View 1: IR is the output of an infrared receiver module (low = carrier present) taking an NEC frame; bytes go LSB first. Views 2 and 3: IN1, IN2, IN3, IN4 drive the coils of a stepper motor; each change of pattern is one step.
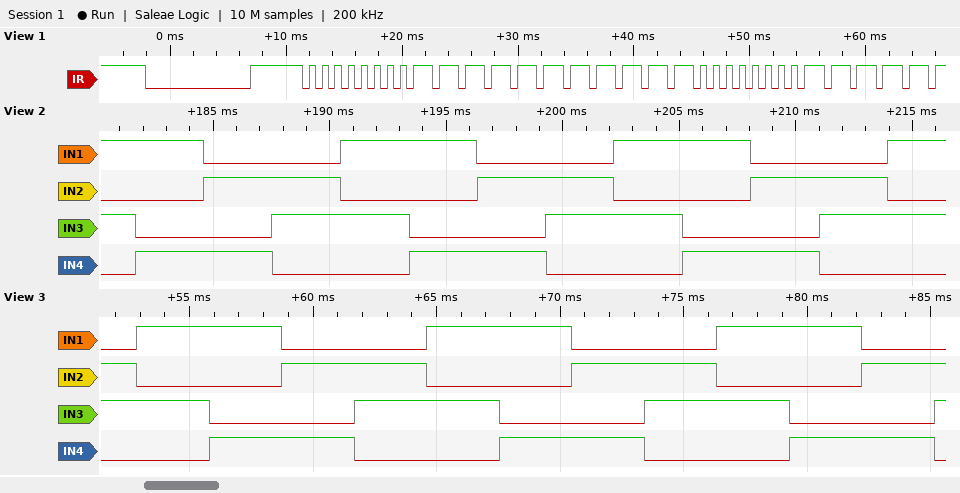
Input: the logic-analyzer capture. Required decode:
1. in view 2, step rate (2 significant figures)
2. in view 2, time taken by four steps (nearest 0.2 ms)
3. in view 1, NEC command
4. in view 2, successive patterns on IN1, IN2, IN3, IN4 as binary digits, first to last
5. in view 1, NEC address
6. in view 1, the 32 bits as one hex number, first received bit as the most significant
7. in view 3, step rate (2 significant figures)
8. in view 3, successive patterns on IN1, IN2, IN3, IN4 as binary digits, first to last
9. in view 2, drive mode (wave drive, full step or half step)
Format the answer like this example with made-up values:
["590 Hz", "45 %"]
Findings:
["340 steps/s", "11.8 ms", "0x07", "1010 1001 0101 0110 1010 1001 0101 0110 1010 1001 0101 0110 1010", "0x00", "0x00FFE01F", "340 steps/s", "0110 1010 1001 0101 0110 1010 1001 0101 0110 1010 1001 0101 0110", "full step"]
